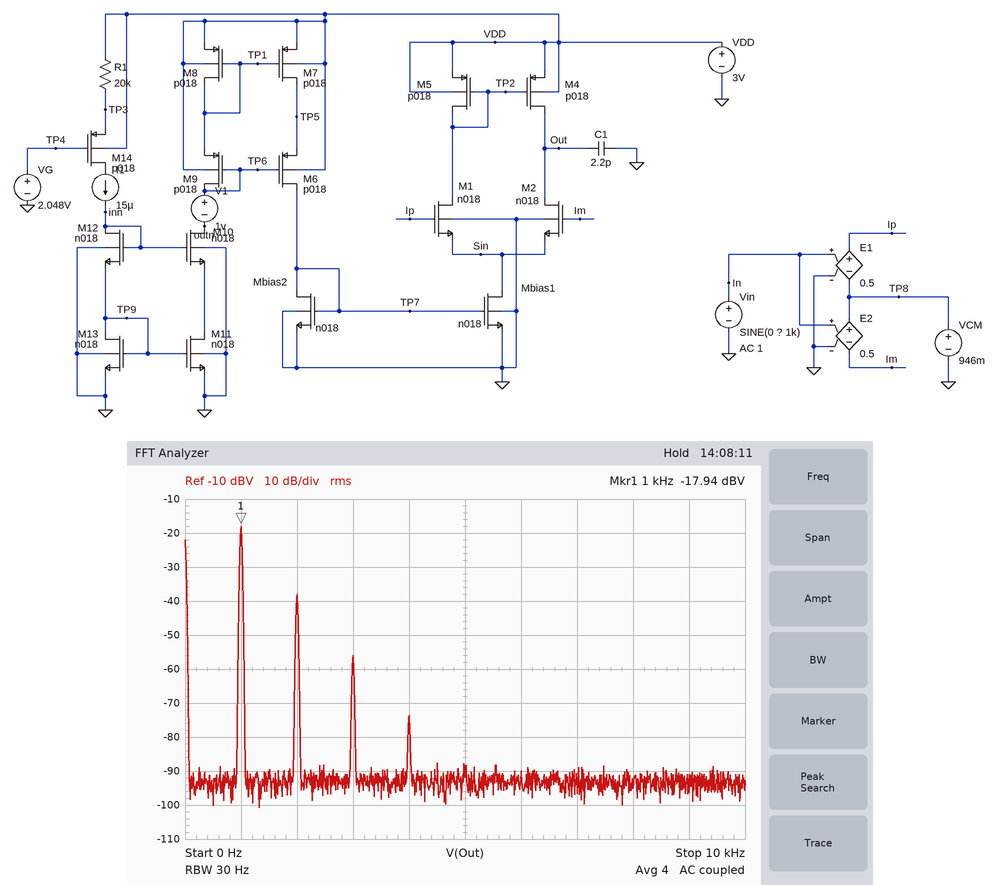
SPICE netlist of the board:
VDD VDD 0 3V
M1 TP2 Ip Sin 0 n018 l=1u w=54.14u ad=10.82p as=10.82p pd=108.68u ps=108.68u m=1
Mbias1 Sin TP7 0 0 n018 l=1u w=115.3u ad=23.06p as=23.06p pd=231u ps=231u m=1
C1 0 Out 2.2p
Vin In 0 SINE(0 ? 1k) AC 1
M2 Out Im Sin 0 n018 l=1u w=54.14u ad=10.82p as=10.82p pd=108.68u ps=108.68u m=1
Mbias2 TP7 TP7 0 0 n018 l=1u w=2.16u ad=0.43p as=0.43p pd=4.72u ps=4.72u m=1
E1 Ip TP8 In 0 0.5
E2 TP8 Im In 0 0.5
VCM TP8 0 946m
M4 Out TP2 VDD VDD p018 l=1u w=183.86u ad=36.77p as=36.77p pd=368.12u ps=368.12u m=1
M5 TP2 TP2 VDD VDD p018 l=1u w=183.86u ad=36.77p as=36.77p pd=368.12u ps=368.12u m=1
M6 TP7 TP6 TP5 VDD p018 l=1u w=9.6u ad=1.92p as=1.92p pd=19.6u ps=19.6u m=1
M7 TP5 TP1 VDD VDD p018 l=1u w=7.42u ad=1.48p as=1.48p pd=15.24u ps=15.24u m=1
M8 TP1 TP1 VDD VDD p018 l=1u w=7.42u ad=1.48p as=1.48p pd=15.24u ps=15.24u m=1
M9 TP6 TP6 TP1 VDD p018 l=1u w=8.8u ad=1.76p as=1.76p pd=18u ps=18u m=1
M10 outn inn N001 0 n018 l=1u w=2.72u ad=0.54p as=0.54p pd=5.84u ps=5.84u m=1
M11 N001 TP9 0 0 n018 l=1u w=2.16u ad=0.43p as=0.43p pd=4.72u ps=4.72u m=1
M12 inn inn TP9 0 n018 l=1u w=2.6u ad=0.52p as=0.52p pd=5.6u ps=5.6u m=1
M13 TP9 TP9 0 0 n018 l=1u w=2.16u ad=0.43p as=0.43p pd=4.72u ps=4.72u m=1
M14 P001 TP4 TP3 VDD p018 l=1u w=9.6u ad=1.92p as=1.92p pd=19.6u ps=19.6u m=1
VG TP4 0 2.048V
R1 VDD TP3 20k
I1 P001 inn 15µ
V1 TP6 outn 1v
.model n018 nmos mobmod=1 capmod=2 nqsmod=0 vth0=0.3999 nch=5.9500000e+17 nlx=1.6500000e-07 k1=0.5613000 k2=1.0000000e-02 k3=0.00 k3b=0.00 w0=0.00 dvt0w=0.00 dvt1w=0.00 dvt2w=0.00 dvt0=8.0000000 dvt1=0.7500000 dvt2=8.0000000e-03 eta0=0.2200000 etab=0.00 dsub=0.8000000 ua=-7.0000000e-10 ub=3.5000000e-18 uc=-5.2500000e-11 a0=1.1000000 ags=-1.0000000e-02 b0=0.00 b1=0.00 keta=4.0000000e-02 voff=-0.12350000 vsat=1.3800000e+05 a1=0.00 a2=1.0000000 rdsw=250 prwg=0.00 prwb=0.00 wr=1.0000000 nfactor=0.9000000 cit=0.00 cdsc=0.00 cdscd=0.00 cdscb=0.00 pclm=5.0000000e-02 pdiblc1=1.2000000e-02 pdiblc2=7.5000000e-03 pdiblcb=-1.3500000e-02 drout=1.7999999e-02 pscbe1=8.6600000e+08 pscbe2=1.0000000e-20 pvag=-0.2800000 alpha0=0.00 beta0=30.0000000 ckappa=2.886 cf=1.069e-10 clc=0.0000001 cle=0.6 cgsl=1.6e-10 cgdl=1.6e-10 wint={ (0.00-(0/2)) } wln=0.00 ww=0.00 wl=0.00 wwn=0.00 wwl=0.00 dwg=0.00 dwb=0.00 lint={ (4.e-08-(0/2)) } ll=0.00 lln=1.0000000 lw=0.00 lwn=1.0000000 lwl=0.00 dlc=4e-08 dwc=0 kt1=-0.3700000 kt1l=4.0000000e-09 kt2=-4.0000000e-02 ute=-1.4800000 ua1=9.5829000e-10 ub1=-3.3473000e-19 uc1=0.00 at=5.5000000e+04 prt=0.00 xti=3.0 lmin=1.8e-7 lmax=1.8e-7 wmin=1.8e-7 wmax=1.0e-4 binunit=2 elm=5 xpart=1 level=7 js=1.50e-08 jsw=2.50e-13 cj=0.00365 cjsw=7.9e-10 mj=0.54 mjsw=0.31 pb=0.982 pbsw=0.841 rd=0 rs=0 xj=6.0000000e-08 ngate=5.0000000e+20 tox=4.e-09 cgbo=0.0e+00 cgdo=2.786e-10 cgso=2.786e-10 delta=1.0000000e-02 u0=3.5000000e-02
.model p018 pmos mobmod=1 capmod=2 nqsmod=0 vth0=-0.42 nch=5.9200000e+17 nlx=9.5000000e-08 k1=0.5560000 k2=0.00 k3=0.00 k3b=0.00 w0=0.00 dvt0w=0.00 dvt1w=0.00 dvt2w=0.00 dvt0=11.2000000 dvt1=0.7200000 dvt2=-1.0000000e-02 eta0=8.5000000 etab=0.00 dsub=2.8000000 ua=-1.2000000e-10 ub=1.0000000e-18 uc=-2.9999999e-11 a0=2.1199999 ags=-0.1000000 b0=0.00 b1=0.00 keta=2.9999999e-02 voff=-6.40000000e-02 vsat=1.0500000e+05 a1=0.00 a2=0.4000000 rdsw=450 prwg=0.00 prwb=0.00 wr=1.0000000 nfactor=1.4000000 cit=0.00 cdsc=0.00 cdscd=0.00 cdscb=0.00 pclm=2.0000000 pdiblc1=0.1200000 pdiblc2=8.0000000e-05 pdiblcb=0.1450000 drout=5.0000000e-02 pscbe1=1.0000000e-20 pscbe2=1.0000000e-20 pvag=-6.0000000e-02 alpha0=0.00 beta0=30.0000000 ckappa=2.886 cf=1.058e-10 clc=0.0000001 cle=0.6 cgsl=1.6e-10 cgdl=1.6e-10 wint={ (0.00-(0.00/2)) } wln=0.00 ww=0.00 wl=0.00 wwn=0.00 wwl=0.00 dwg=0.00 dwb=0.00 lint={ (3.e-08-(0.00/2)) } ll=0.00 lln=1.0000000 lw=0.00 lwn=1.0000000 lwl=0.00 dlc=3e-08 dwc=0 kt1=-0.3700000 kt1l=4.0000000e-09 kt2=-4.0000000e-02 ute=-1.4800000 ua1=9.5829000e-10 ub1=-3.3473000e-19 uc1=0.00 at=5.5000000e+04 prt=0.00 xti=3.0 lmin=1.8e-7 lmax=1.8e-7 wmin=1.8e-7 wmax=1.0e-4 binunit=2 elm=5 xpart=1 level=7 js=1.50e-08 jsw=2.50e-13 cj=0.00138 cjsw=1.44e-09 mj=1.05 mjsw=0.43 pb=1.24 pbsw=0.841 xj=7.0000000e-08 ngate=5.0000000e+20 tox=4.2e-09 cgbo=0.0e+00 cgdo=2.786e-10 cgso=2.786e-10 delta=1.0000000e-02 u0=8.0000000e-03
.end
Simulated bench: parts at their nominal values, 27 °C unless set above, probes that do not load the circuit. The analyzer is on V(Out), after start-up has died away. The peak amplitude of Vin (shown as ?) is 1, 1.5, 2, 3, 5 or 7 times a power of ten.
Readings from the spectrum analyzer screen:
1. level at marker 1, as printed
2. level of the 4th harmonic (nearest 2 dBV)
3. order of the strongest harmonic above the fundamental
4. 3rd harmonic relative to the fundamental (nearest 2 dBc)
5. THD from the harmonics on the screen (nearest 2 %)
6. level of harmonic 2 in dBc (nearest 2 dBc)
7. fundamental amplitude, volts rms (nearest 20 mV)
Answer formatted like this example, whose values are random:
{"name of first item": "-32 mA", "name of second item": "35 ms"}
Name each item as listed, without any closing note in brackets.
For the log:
{"level at marker 1, as printed": "-17.94 dBV", "level of the 4th harmonic": "-74 dBV", "order of the strongest harmonic above the fundamental": "2", "3rd harmonic relative to the fundamental": "-38 dBc", "THD from the harmonics on the screen": "10 %", "level of harmonic 2 in dBc": "-20 dBc", "fundamental amplitude, volts rms": "120 mV"}
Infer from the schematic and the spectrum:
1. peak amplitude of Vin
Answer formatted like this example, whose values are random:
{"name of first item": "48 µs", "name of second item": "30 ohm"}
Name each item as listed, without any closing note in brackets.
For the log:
{"peak amplitude of Vin": "5 mV"}
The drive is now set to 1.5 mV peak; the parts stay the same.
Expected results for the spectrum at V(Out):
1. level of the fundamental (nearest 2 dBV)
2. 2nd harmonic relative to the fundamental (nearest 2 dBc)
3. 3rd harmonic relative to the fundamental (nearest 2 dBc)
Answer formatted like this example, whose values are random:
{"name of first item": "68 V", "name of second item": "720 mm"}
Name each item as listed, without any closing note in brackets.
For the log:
{"level of the fundamental": "-28 dBV", "2nd harmonic relative to the fundamental": "-30 dBc", "3rd harmonic relative to the fundamental": "-60 dBc"}
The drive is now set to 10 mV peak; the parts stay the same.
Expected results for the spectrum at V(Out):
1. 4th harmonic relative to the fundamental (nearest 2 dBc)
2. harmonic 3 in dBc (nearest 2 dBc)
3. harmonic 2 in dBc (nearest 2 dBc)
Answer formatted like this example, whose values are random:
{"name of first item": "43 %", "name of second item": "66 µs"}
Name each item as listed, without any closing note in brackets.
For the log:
{"4th harmonic relative to the fundamental": "-42 dBc", "harmonic 3 in dBc": "-26 dBc", "harmonic 2 in dBc": "-14 dBc"}
